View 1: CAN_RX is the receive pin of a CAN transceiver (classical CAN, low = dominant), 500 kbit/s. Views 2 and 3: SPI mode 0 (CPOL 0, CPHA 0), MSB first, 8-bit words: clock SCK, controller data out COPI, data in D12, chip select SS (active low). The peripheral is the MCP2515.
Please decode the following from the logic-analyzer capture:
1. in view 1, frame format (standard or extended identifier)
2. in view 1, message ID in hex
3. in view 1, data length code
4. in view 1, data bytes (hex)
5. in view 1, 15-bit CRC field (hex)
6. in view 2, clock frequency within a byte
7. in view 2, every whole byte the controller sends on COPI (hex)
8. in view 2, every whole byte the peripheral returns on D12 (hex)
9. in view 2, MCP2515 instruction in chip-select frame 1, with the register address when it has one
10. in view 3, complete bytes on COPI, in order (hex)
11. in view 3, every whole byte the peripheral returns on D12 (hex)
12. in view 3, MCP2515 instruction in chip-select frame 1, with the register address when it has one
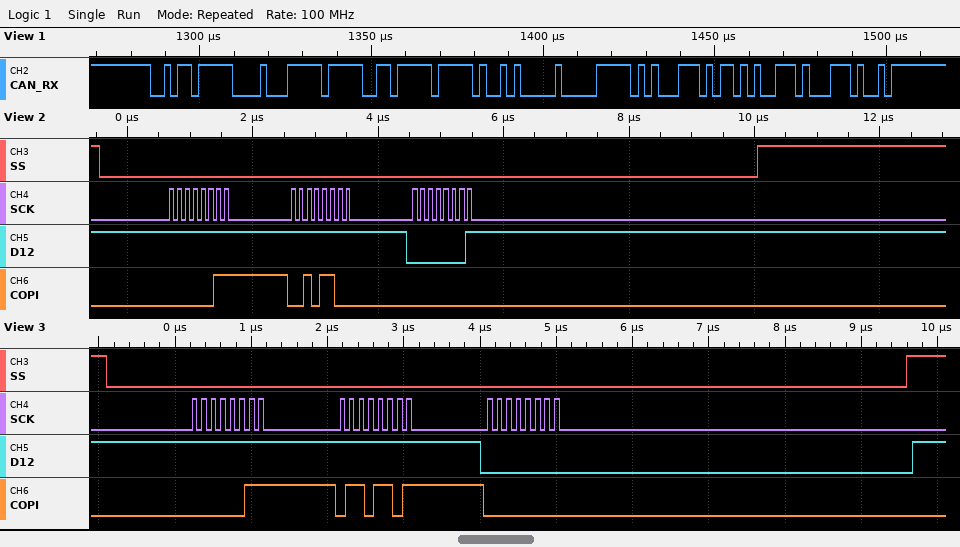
standard
0x2DF
8
FF DB FF 94 00 FA 3A D4
0x7474
8 MHz
03 2C 00
FF FF 01
READ 0x2C
03 6D 00
FF FF 00
READ 0x6D
